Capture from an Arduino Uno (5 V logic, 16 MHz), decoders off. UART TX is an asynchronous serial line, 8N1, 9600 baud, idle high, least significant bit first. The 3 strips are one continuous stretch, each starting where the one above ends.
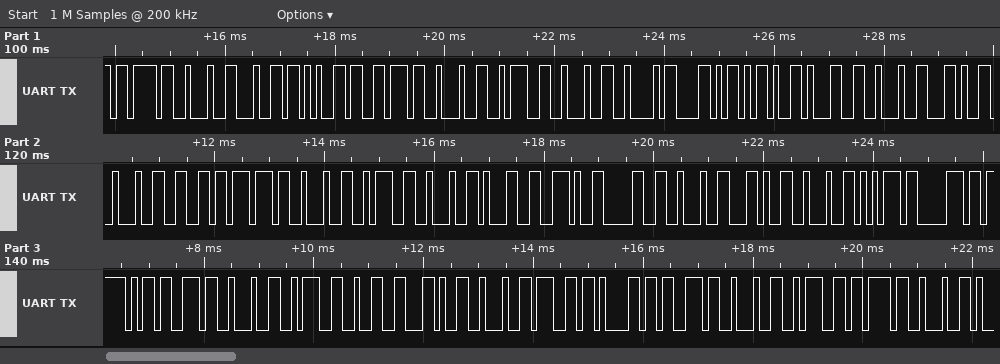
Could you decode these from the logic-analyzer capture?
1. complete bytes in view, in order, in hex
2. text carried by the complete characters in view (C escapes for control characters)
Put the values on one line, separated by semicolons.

7B 22 64 65 76 22 3A 22 42 58 2D 31 22 2C 22 66 77 22 3A 22 31 2E 30 22 2C 22 75 70 5F 73 22 3A 32 2C 22 67 61 73 22 3A 7B 22; "{\"dev\":\"BX-1\",\"fw\":\"1.0\",\"up_s\":2,\"gas\":{\""
